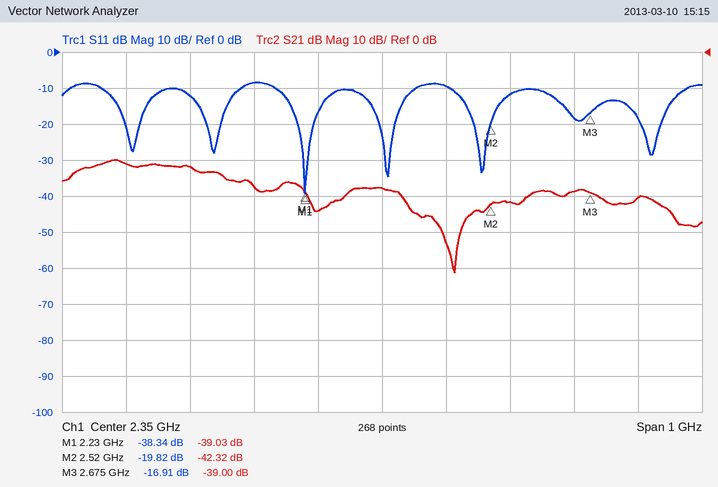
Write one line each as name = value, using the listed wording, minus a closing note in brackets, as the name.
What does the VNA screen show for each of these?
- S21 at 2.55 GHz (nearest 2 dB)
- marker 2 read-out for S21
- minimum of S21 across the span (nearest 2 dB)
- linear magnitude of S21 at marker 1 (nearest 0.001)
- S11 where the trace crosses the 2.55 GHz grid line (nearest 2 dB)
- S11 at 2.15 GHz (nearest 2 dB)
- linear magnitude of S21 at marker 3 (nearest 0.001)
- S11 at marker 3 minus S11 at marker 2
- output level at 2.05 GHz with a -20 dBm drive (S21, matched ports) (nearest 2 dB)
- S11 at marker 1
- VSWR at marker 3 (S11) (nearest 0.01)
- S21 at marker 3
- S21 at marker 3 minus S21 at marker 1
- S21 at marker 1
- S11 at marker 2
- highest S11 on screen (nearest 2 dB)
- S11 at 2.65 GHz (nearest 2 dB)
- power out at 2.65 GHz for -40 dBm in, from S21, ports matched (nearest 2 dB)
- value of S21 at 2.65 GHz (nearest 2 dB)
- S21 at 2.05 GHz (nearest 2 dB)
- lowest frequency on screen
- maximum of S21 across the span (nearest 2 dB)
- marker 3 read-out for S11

S21 at 2.55 GHz = -42 dB
marker 2 read-out for S21 = -42.32 dB
minimum of S21 across the span = -62 dB
linear magnitude of S21 at marker 1 = 0.011
S11 where the trace crosses the 2.55 GHz grid line = -12 dB
S11 at 2.15 GHz = -8 dB
linear magnitude of S21 at marker 3 = 0.011
S11 at marker 3 minus S11 at marker 2 = 2.91 dB
output level at 2.05 GHz with a -20 dBm drive (S21, matched ports) = -52 dBm
S11 at marker 1 = -38.34 dB
VSWR at marker 3 (S11) = 1.33
S21 at marker 3 = -39.00 dB
S21 at marker 3 minus S21 at marker 1 = 0.03 dB
S21 at marker 1 = -39.03 dB
S11 at marker 2 = -19.82 dB
highest S11 on screen = -8 dB
S11 at 2.65 GHz = -18 dB
power out at 2.65 GHz for -40 dBm in, from S21, ports matched = -78 dBm
value of S21 at 2.65 GHz = -38 dB
S21 at 2.05 GHz = -32 dB
lowest frequency on screen = 1.85 GHz
maximum of S21 across the span = -30 dB
marker 3 read-out for S11 = -16.91 dB
